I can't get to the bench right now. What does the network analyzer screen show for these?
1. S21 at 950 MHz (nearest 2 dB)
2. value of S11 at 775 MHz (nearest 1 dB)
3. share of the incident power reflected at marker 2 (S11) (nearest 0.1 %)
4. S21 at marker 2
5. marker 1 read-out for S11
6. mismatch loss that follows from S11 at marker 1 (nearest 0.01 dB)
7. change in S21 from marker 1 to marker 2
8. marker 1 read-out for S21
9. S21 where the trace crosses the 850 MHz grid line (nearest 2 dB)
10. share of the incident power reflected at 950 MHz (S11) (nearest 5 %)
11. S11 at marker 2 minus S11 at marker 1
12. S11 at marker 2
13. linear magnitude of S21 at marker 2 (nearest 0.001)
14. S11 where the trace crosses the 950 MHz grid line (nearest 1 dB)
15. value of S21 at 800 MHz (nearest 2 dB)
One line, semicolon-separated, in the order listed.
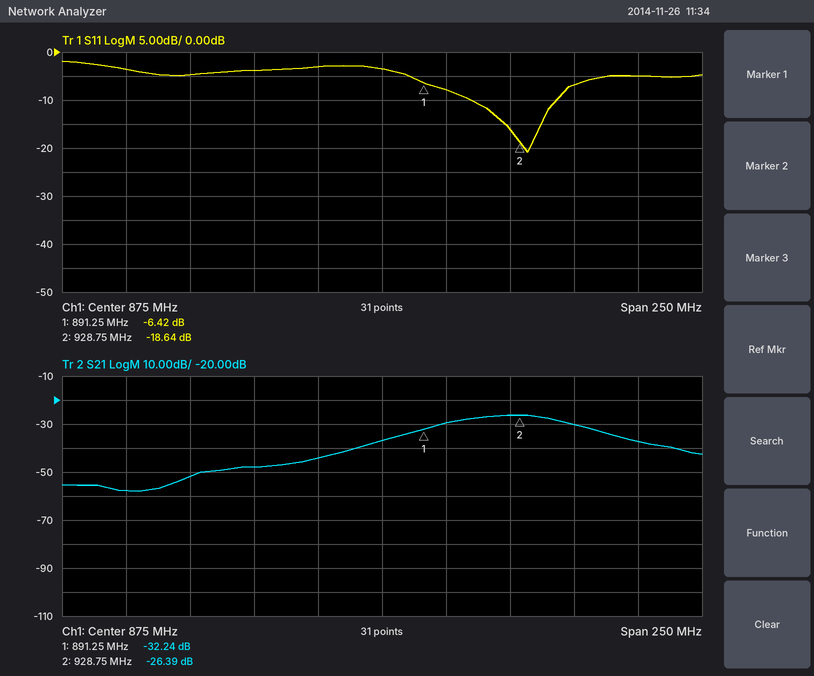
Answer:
-30 dB; -4 dB; 1.4 %; -26.39 dB; -6.42 dB; 1.12 dB; 5.85 dB; -32.24 dB; -44 dB; 20 %; -12.22 dB; -18.64 dB; 0.048; -7 dB; -52 dB
